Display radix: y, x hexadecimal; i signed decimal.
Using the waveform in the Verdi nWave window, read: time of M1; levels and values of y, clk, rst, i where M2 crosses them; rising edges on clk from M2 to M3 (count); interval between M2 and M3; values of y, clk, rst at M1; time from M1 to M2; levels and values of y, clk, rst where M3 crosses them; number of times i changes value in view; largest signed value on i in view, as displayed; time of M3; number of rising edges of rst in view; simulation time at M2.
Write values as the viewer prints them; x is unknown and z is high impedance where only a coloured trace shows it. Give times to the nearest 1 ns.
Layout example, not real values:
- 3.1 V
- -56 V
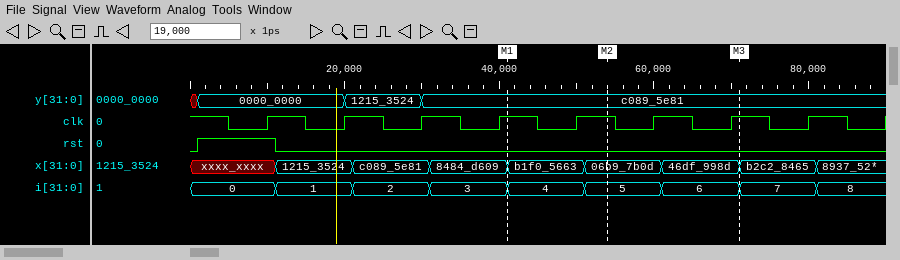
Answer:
- 41 ns
- y=c089_5e81, clk=1, rst=0, i=5
- 2
- 17 ns
- y=c089_5e81, clk=1, rst=0
- 13 ns
- y=c089_5e81, clk=1, rst=0
- 8
- 8
- 71 ns
- 1
- 54 ns
